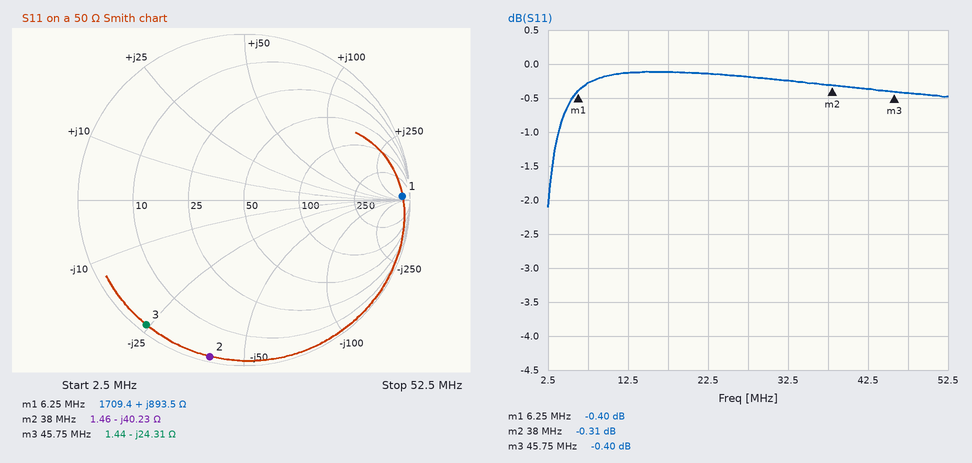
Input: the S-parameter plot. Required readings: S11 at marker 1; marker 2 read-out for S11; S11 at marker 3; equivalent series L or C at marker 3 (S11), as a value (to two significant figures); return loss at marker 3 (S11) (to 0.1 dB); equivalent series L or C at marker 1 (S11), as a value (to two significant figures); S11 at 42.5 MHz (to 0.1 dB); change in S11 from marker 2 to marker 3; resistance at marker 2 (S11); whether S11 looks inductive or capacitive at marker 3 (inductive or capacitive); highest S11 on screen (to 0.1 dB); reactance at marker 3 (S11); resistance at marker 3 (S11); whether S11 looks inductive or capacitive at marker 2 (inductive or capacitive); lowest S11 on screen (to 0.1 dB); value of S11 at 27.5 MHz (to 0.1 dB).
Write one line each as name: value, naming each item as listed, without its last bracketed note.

S11 at marker 1: -0.40 dB
marker 2 read-out for S11: -0.31 dB
S11 at marker 3: -0.40 dB
equivalent series L or C at marker 3 (S11), as a value: 140 pF
return loss at marker 3 (S11): 0.4 dB
equivalent series L or C at marker 1 (S11), as a value: 23 µH
S11 at 42.5 MHz: -0.4 dB
change in S11 from marker 2 to marker 3: -0.09 dB
resistance at marker 2: 1.46 Ω
whether S11 looks inductive or capacitive at marker 3: capacitive
highest S11 on screen: -0.1 dB
reactance at marker 3: -24.31 Ω
resistance at marker 3: 1.44 Ω
whether S11 looks inductive or capacitive at marker 2: capacitive
lowest S11 on screen: -2.1 dB
value of S11 at 27.5 MHz: -0.2 dB
